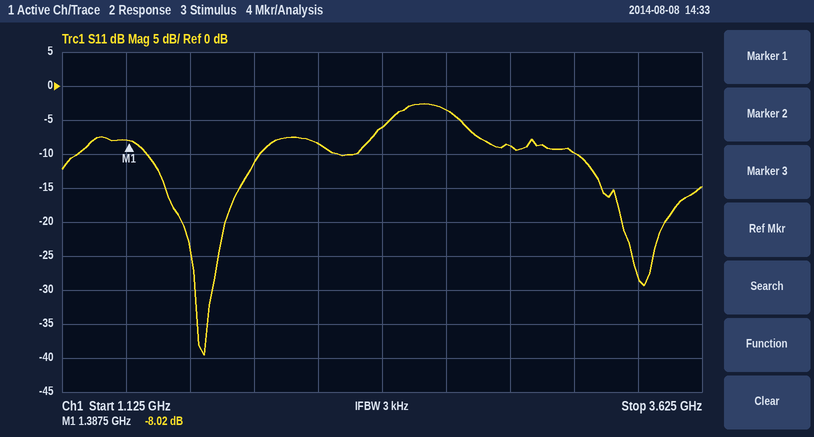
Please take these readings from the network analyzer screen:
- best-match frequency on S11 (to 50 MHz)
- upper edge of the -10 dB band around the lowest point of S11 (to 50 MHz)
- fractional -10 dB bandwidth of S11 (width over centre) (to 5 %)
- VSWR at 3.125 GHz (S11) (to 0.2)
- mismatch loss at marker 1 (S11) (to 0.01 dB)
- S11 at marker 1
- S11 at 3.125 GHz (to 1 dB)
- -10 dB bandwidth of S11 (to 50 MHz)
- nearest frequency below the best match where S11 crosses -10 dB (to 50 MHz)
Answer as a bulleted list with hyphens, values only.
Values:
- 1.70 GHz
- 1.90 GHz
- 25 %
- 2.0
- 0.75 dB
- -8.02 dB
- -10 dB
- 450 MHz
- 1.45 GHz
